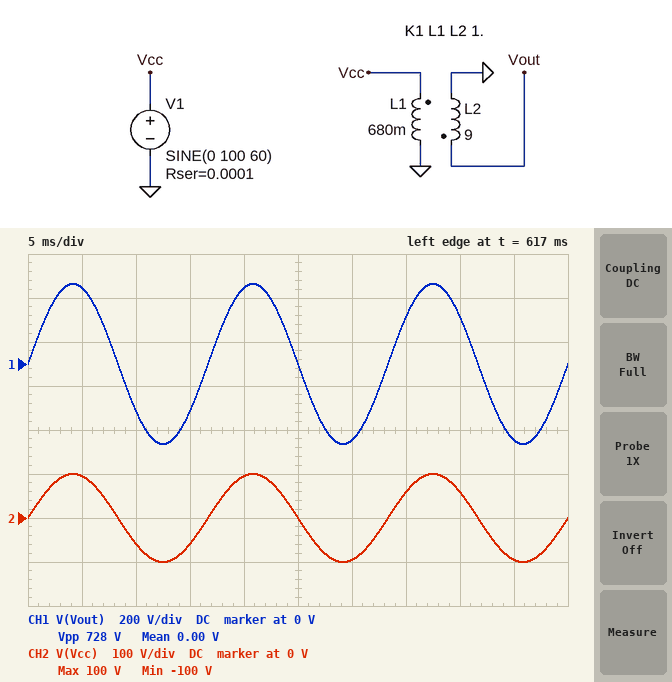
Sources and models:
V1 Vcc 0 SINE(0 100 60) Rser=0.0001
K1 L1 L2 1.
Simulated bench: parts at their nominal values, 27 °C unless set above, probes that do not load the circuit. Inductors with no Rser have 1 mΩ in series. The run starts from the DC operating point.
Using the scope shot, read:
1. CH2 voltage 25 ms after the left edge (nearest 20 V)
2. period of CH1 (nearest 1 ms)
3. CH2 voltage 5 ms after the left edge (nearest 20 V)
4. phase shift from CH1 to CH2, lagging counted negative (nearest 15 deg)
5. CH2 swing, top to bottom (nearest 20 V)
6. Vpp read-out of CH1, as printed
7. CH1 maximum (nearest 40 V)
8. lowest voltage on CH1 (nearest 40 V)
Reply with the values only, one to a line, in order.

0 V
17 ms
100 V
0 deg
200 V
728 V
360 V
-360 V
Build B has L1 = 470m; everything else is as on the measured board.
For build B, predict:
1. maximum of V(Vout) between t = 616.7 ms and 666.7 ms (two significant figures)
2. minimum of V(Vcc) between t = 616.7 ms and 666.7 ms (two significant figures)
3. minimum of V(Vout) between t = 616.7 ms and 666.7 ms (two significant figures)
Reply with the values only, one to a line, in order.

440 V
-100 V
-440 V
